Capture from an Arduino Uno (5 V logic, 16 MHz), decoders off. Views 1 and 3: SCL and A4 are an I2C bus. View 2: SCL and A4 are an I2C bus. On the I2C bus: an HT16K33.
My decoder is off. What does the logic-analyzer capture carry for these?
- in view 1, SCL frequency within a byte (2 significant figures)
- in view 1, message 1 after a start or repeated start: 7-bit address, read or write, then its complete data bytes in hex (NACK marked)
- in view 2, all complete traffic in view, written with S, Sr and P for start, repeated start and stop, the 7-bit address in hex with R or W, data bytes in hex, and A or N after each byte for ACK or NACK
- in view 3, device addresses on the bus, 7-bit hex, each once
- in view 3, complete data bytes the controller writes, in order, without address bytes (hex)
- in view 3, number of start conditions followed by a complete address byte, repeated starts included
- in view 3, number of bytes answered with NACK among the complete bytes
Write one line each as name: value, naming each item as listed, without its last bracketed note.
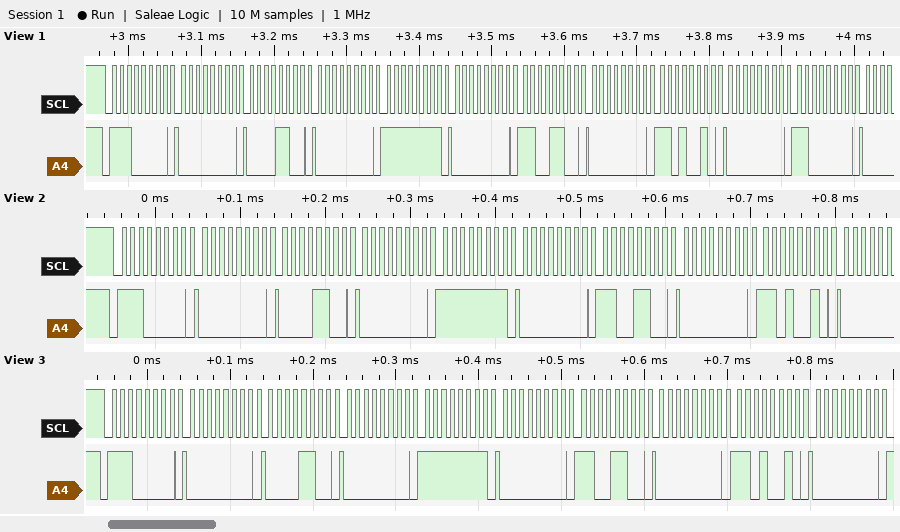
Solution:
in view 1, SCL frequency within a byte: 100 kHz
in view 1, message 1 after a start or repeated start: 7-bit address, read or write, then its complete data bytes in hex: 0x70 write: 00 0C 00 FF 00 CC 00 D2 00 C0
in view 2, all complete traffic in view, written with S, Sr and P for start, repeated start and stop, the 7-bit address in hex with R or W, data bytes in hex, and A or N after each byte for ACK or NACK: S 70W A 00 A 0C A 00 A FF A 00 A CC A 00 A D2 A
in view 3, device addresses on the bus, 7-bit hex, each once: 0x70
in view 3, complete data bytes the controller writes, in order, without address bytes: 00 0C 00 FF 00 CC 00 D2 00
in view 3, number of start conditions followed by a complete address byte, repeated starts included: 1
in view 3, number of bytes answered with NACK among the complete bytes: 0
